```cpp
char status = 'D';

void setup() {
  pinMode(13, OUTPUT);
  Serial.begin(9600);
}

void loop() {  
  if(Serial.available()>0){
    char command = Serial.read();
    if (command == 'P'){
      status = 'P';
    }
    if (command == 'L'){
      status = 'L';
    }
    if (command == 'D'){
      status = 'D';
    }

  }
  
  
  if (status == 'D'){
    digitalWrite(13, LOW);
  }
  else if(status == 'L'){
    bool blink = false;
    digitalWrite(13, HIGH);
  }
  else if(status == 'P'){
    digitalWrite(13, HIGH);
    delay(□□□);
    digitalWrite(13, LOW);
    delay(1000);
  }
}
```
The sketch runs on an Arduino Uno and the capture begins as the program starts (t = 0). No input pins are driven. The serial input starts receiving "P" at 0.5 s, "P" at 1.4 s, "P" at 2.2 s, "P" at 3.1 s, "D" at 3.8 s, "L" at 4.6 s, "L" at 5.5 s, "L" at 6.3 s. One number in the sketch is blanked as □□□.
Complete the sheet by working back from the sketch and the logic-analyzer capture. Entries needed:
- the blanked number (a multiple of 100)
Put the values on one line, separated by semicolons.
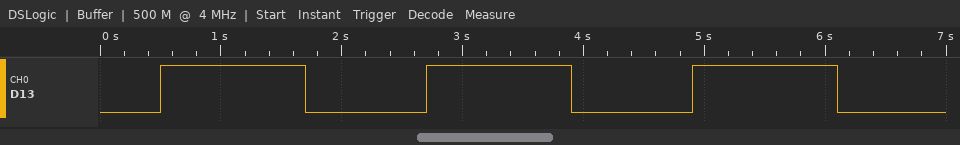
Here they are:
1200
